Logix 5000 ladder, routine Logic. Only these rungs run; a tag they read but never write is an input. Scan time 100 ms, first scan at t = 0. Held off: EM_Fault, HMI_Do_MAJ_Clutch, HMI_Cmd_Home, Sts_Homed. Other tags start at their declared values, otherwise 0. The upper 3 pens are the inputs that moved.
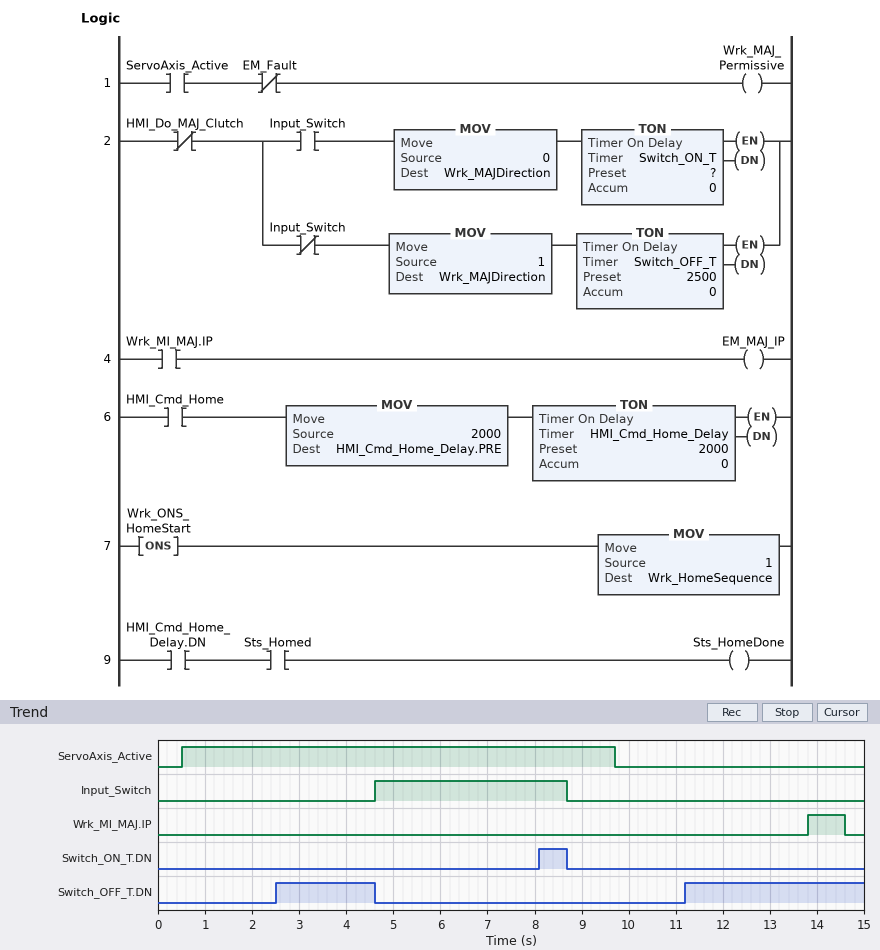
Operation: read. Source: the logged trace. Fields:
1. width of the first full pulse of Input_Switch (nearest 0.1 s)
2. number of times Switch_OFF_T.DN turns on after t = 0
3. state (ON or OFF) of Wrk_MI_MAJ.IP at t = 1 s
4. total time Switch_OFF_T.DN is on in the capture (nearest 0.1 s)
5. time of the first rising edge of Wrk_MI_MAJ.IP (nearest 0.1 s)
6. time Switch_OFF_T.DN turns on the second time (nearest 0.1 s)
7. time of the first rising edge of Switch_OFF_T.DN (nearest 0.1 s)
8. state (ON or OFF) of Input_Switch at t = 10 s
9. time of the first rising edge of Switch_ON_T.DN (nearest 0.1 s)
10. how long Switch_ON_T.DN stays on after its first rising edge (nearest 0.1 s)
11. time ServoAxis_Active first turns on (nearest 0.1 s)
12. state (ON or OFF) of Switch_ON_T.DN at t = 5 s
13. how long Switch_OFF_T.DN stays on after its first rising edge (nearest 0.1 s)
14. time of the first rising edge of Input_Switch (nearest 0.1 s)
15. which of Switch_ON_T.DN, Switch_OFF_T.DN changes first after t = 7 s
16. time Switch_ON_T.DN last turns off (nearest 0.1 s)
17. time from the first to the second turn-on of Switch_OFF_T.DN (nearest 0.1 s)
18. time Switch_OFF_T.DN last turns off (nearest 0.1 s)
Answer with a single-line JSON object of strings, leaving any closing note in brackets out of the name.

{"width of the first full pulse of Input_Switch": "4.1 s", "number of times Switch_OFF_T.DN turns on after t = 0": "2", "state (ON or OFF) of Wrk_MI_MAJ.IP at t = 1 s": "OFF", "total time Switch_OFF_T.DN is on in the capture": "5.9 s", "time of the first rising edge of Wrk_MI_MAJ.IP": "13.8 s", "time Switch_OFF_T.DN turns on the second time": "11.2 s", "time of the first rising edge of Switch_OFF_T.DN": "2.5 s", "state (ON or OFF) of Input_Switch at t = 10 s": "OFF", "time of the first rising edge of Switch_ON_T.DN": "8.1 s", "how long Switch_ON_T.DN stays on after its first rising edge": "0.6 s", "time ServoAxis_Active first turns on": "0.5 s", "state (ON or OFF) of Switch_ON_T.DN at t = 5 s": "OFF", "how long Switch_OFF_T.DN stays on after its first rising edge": "2.1 s", "time of the first rising edge of Input_Switch": "4.6 s", "which of Switch_ON_T.DN, Switch_OFF_T.DN changes first after t = 7 s": "Switch_ON_T.DN", "time Switch_ON_T.DN last turns off": "8.7 s", "time from the first to the second turn-on of Switch_OFF_T.DN": "8.7 s", "time Switch_OFF_T.DN last turns off": "4.6 s"}
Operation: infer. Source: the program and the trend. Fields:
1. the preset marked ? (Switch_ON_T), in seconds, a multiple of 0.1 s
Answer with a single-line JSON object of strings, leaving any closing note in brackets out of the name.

{"the preset marked ? (Switch_ON_T), in seconds, a multiple of 0.1 s": "3.5 s"}
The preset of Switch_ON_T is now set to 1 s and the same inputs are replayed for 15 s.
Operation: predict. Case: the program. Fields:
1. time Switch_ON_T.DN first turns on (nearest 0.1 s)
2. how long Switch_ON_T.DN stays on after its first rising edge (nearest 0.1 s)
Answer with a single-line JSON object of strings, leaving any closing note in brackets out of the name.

{"time Switch_ON_T.DN first turns on": "5.6 s", "how long Switch_ON_T.DN stays on after its first rising edge": "3.1 s"}
